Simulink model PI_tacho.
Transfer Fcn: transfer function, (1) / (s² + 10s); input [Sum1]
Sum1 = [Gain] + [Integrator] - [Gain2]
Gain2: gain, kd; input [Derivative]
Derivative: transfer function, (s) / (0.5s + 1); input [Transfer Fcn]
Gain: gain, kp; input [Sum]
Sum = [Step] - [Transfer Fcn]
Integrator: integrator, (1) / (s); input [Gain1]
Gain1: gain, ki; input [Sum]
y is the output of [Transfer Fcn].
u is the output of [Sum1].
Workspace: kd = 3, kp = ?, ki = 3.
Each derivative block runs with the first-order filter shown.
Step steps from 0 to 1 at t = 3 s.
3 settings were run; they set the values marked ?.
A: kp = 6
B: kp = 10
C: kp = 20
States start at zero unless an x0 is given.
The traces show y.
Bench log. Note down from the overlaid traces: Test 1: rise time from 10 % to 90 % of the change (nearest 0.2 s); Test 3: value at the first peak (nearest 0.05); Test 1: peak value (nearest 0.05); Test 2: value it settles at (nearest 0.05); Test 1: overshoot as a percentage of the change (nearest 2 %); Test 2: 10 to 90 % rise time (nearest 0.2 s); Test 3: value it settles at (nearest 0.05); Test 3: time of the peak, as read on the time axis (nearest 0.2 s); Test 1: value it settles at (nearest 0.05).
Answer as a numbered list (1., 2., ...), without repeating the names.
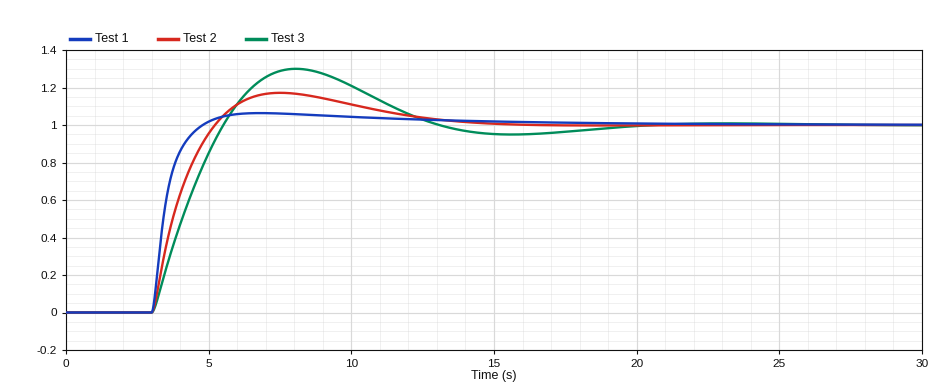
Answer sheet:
1. 1.0 s
2. 1.30
3. 1.05
4. 1.00
5. 6 %
6. 1.6 s
7. 1.00
8. 8.0 s
9. 1.00
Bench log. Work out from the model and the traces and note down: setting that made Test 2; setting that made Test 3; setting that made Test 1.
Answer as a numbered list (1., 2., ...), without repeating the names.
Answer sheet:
1. B
2. A
3. C
